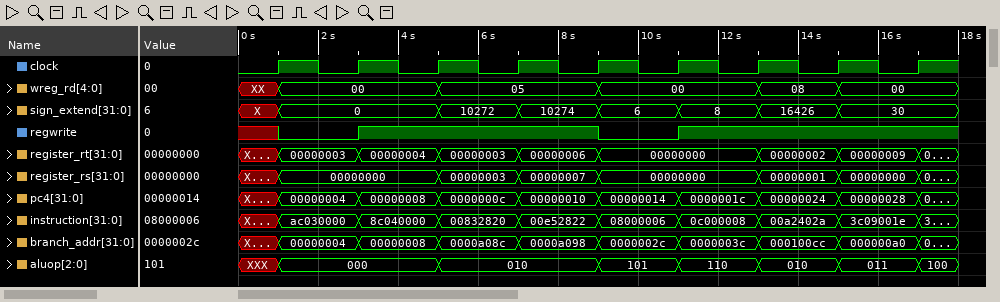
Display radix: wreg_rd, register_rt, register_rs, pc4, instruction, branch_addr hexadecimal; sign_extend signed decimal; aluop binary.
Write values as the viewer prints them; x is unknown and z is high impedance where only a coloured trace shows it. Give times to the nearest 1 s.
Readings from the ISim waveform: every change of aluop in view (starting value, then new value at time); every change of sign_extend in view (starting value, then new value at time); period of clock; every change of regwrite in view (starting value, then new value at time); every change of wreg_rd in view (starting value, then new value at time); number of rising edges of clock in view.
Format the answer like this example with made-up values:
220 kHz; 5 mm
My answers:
XXX, 000 at 1 s, 010 at 5 s, 101 at 9 s, 110 at 11 s, 010 at 13 s, 011 at 15 s, 100 at 17 s; X, 0 at 1 s, 10272 at 5 s, 10274 at 7 s, 6 at 9 s, 8 at 11 s, 16426 at 13 s, 30 at 15 s; 2 s; x, 0 at 1 s, 1 at 3 s, 0 at 9 s, 1 at 11 s; XX, 00 at 1 s, 05 at 5 s, 00 at 9 s, 08 at 13 s, 00 at 15 s; 9
